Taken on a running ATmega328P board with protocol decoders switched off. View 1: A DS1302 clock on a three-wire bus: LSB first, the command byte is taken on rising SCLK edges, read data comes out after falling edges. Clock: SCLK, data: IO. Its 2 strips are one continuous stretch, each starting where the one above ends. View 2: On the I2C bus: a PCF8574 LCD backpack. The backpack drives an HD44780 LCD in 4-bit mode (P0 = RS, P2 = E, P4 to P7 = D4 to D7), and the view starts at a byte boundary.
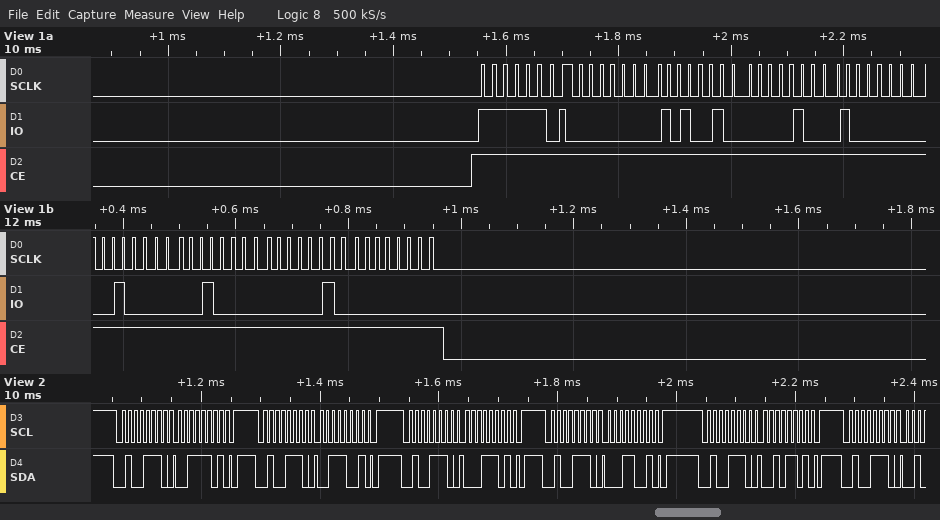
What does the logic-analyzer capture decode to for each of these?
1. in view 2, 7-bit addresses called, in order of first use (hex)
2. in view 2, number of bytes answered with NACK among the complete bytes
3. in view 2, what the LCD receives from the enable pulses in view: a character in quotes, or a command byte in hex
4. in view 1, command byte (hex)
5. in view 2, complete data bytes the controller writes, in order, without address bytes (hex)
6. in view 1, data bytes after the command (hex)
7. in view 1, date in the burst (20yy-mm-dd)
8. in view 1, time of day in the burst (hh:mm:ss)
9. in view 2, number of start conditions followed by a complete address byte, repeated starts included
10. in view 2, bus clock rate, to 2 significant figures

0x27
0
'1'
0xBF
3D 39 1D 19 2D
00 25 10 01 04 04 20 00
2020-04-01
10:25:00
6
100 kHz
